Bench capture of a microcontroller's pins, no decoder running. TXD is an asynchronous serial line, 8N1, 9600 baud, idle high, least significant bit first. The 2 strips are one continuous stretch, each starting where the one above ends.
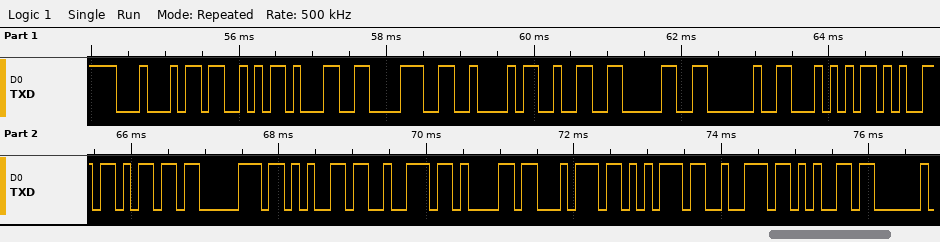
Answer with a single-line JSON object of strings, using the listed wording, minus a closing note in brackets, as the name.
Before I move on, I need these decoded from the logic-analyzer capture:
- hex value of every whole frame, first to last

{"hex value of every whole frame, first to last": "44 53 31 38 42 32 30 20 54 65 6D 70 65 72 61 74 75 72 65"}
